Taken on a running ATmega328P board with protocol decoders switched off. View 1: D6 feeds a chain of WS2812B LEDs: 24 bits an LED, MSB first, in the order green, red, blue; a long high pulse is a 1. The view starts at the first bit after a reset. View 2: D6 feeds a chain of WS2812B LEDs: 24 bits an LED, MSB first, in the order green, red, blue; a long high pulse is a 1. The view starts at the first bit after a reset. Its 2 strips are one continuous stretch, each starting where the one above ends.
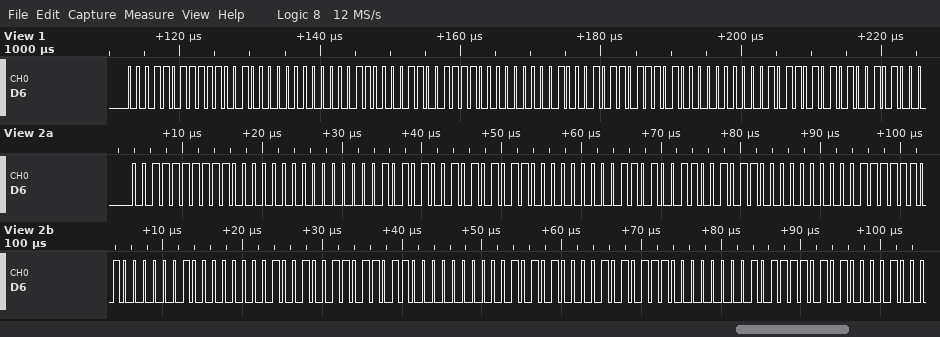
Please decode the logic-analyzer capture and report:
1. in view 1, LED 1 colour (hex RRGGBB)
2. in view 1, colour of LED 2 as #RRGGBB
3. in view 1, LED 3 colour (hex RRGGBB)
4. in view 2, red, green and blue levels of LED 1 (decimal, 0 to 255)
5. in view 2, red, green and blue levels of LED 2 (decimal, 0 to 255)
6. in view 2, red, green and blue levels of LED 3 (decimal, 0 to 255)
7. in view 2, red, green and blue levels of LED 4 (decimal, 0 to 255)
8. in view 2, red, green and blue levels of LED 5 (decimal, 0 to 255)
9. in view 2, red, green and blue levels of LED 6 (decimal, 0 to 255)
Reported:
#E41B00
#CF3000
#BA4500
192, 63, 0
171, 84, 0
150, 105, 0
129, 126, 0
108, 147, 0
87, 168, 0
